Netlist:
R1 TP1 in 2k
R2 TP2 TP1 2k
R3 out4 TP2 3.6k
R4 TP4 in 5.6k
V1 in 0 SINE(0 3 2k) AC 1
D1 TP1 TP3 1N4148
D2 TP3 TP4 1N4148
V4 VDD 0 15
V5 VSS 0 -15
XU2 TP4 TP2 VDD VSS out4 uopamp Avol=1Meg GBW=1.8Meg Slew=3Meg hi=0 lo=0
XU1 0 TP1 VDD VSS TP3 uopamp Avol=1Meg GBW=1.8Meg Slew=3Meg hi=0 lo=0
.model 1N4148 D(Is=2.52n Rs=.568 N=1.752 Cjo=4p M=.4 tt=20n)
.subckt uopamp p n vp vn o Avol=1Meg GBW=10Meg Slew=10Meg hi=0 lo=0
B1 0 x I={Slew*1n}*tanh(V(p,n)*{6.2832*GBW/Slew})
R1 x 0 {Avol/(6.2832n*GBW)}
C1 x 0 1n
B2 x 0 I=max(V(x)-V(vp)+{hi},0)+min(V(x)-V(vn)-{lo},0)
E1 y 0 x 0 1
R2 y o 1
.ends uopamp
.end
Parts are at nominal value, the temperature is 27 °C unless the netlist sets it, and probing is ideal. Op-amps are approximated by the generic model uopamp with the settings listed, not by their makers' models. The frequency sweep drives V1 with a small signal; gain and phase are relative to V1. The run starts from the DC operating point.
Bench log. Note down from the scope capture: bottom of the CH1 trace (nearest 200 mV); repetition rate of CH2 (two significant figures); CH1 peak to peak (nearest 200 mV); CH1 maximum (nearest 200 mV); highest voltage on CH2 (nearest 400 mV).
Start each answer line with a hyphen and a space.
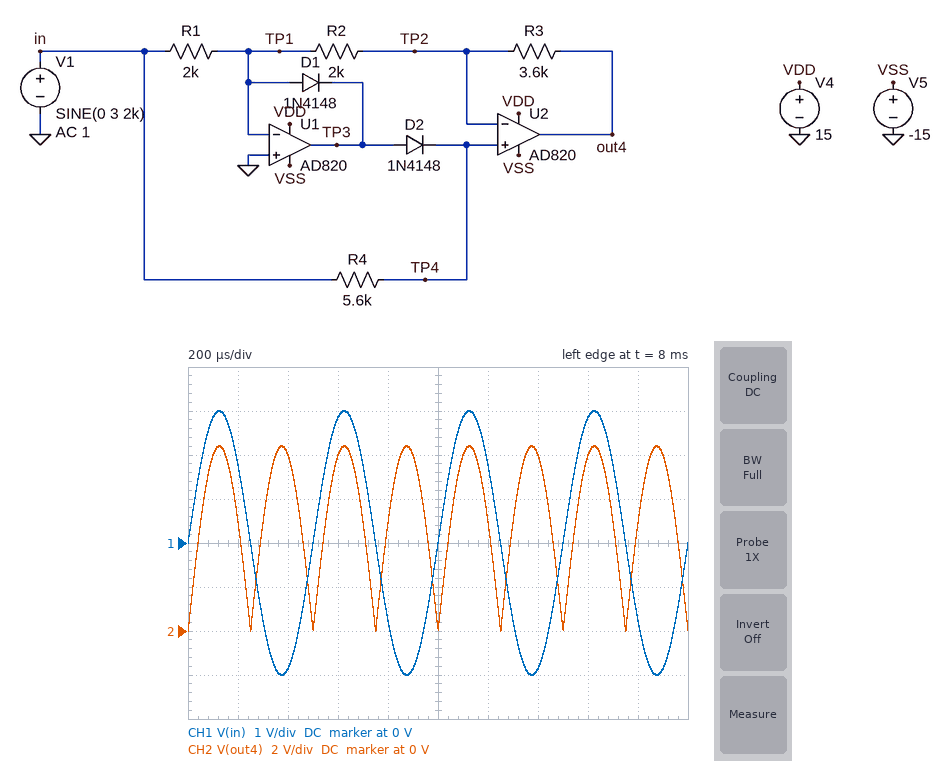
- -3.0 V
- 4.0 kHz
- 6.0 V
- 3.0 V
- 8.4 V
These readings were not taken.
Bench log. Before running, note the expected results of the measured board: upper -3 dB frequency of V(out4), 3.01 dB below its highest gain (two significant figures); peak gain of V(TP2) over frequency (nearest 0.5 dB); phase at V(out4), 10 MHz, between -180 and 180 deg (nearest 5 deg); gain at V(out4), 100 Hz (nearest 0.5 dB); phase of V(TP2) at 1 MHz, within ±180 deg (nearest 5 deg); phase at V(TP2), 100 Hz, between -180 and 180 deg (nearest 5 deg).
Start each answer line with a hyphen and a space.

- 460 Hz
- -2.0 dB
- 165 deg
- 2.0 dB
- -20 deg
- 135 deg
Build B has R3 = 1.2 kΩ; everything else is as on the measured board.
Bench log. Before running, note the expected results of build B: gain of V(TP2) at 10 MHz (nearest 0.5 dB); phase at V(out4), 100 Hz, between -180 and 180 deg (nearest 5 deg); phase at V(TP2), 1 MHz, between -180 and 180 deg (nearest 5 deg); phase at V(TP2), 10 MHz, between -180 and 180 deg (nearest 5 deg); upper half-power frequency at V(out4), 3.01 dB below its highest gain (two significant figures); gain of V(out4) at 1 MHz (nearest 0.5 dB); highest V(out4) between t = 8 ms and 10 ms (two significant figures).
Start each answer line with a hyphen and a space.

- -15.0 dB
- 145 deg
- -30 deg
- -25 deg
- 1.5 MHz
- -4.0 dB
- 4.8 V
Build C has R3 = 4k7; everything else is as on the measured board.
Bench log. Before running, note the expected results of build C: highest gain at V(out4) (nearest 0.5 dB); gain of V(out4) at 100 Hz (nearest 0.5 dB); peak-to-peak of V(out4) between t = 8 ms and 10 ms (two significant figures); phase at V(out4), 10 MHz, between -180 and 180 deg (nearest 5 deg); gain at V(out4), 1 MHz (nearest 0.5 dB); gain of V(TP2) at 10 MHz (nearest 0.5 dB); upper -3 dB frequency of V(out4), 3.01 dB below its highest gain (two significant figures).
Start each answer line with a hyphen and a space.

- 4.0 dB
- 3.5 dB
- 10 V
- 150 deg
- -7.5 dB
- -7.0 dB
- 390 Hz
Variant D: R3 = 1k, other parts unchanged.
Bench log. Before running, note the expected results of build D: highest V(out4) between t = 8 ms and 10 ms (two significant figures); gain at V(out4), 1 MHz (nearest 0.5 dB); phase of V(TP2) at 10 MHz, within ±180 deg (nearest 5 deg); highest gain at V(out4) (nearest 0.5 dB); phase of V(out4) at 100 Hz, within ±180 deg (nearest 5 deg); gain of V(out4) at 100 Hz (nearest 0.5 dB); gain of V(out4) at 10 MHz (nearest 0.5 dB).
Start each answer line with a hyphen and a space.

- 4.5 V
- -4.0 dB
- -30 deg
- -2.5 dB
- 145 deg
- -3.0 dB
- -23.5 dB
